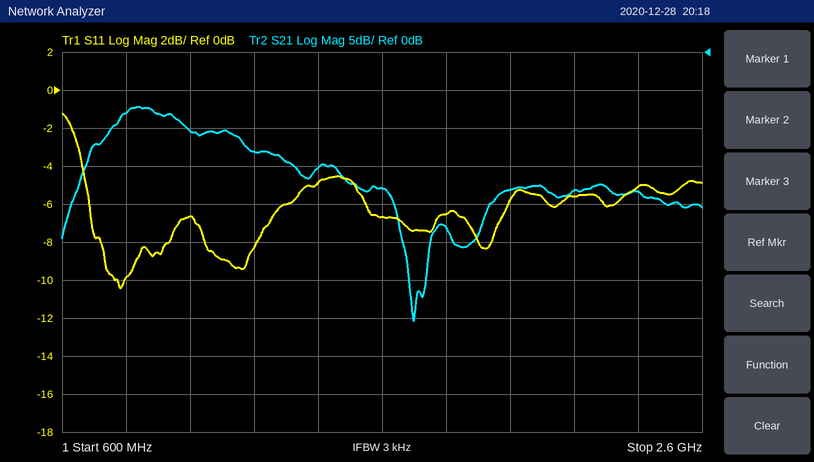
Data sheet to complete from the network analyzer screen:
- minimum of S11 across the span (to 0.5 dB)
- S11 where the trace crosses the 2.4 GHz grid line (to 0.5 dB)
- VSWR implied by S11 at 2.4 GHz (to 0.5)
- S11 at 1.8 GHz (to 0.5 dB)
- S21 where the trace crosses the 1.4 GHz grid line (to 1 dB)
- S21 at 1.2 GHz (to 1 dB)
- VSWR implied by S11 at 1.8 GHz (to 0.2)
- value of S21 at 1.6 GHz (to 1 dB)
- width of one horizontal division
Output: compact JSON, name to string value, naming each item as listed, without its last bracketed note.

{"minimum of S11 across the span": "-10.5 dB", "S11 where the trace crosses the 2.4 GHz grid line": "-5.0 dB", "VSWR implied by S11 at 2.4 GHz": "3.5", "S11 at 1.8 GHz": "-6.5 dB", "S21 where the trace crosses the 1.4 GHz grid line": "-15 dB", "S21 at 1.2 GHz": "-13 dB", "VSWR implied by S11 at 1.8 GHz": "2.8", "value of S21 at 1.6 GHz": "-18 dB", "width of one horizontal division": "200 MHz"}
